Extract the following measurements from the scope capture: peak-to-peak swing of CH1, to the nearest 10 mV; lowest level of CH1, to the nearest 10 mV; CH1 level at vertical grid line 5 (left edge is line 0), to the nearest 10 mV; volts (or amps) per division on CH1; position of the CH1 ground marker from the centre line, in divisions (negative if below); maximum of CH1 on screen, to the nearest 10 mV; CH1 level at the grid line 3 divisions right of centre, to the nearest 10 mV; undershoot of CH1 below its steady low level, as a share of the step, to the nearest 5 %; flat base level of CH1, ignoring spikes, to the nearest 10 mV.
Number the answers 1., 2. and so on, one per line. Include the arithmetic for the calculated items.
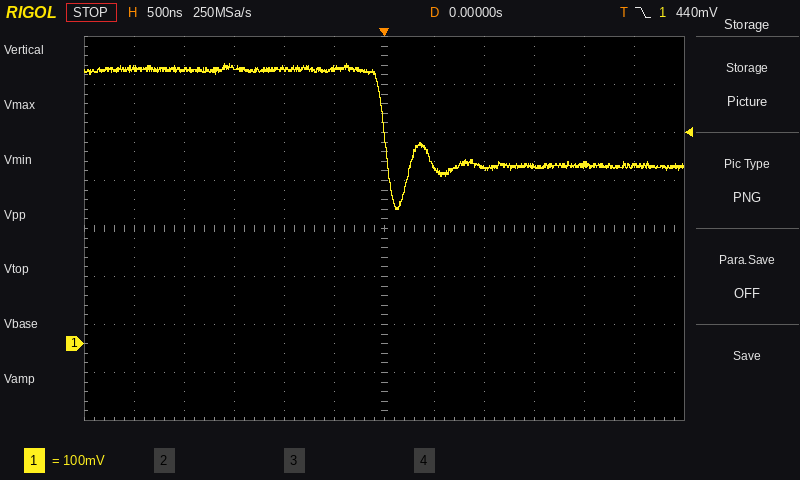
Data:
1. 580 mV − (280 mV) = 300 mV
2. 280 mV
3. 570 mV
4. 100 mV
5. -2.4 div
6. 580 mV
7. 370 mV
8. 45 %
9. 370 mV
